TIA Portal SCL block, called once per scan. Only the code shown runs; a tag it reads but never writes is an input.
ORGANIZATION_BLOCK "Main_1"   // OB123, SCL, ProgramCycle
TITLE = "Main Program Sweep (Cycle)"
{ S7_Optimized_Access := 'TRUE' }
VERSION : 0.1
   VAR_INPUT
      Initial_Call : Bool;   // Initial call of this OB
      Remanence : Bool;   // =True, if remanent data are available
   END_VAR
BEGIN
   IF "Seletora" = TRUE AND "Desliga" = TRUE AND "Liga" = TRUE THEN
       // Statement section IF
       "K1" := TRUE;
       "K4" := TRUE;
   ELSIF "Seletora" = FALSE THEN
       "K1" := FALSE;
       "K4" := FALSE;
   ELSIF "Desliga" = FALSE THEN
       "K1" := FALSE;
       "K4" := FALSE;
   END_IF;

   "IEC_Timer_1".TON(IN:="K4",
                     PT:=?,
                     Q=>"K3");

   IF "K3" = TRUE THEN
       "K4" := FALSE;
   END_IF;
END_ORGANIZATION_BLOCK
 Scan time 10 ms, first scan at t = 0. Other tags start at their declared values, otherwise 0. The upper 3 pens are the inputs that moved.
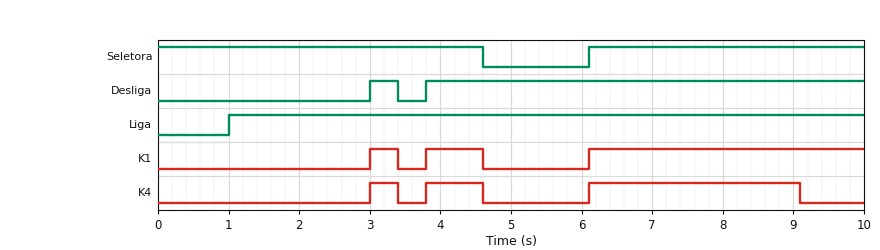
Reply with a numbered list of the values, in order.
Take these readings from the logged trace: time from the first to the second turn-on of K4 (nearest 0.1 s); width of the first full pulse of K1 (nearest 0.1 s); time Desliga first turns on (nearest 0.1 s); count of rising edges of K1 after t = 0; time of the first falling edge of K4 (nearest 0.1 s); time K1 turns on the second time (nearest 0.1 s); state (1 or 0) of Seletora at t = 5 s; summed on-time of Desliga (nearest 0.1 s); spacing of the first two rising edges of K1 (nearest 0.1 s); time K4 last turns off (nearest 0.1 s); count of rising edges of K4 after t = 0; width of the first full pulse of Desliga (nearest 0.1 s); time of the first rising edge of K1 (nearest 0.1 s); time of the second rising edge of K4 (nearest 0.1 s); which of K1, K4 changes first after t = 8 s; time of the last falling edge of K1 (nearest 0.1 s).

1. 0.8 s
2. 0.4 s
3. 3.0 s
4. 3
5. 3.4 s
6. 3.8 s
7. 0
8. 6.6 s
9. 0.8 s
10. 9.1 s
11. 3
12. 0.4 s
13. 3.0 s
14. 3.8 s
15. K4
16. 4.6 s
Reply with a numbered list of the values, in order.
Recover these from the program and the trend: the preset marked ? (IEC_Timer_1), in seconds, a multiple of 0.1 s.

1. 3.0 s
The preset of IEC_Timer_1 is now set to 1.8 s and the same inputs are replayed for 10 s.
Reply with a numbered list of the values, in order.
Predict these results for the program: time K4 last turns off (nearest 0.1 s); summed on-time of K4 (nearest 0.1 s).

1. 7.9 s
2. 3.0 s
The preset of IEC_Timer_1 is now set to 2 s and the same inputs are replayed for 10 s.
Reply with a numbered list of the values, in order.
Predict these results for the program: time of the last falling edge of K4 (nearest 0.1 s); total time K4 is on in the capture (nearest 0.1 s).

1. 8.1 s
2. 3.2 s
